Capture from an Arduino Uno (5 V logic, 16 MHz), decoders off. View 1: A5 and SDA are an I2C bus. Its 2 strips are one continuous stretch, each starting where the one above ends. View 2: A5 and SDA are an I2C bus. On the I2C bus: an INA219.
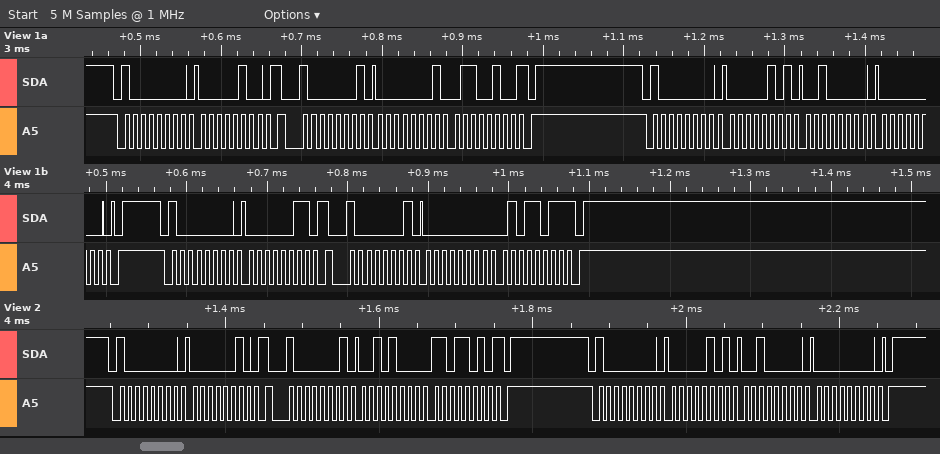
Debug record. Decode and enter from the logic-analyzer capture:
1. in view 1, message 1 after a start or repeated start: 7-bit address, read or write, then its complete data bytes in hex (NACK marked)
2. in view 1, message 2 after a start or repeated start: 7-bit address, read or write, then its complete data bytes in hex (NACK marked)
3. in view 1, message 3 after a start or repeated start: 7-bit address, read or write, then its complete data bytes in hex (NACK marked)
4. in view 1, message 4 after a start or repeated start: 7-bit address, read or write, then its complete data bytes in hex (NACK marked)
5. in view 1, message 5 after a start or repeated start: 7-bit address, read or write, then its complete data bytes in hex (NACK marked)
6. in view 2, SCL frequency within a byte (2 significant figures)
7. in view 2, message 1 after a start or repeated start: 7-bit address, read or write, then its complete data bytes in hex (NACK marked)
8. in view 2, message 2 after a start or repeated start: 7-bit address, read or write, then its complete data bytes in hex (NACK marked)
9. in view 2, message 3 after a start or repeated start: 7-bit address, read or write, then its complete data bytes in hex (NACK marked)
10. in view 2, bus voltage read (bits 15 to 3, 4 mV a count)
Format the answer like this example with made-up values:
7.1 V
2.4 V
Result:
0x40 write: 04
0x40 read: 01 64 NACK
0x40 write: 05 20 00
0x40 write: 03
0x40 read: 00 5B NACK
100 kHz
0x40 write: 02
0x40 read: 28 DA NACK
0x40 write: 05 20 00
5.228 V
